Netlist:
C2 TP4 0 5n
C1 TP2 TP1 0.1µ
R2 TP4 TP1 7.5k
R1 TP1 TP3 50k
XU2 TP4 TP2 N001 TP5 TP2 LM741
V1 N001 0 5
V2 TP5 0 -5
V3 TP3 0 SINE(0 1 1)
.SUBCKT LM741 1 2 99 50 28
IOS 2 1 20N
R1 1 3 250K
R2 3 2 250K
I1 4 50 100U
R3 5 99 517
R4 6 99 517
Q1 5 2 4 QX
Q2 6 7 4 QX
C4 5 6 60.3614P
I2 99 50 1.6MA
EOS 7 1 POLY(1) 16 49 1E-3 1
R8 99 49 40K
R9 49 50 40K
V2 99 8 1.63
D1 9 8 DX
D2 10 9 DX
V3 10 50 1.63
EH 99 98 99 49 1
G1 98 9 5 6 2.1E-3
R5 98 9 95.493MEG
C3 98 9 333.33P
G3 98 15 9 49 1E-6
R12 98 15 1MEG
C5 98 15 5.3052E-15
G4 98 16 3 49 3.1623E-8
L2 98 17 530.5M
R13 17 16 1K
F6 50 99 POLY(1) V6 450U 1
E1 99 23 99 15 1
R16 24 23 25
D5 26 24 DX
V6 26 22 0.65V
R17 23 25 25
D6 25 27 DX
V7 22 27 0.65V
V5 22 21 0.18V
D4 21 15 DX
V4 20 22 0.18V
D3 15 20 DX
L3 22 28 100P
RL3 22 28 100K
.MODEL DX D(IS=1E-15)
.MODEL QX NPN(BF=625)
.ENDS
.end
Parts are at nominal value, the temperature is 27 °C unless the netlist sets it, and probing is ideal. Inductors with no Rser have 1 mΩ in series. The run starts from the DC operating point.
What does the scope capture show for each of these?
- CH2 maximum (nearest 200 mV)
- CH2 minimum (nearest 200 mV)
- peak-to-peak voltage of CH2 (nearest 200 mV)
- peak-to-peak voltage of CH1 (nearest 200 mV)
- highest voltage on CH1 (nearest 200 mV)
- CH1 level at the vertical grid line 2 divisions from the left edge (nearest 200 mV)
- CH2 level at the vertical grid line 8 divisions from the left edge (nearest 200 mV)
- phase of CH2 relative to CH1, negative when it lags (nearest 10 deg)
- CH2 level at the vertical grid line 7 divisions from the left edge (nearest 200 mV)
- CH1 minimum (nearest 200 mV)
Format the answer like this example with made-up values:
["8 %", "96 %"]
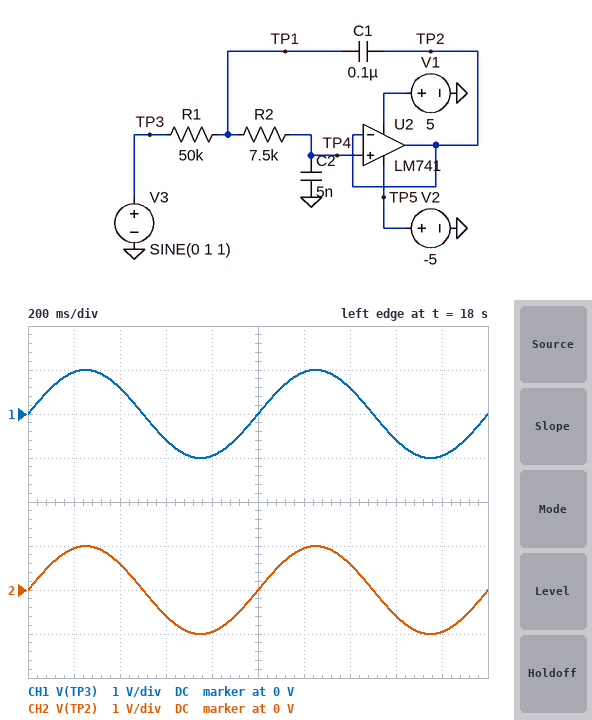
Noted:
["1.0 V", "-1.0 V", "2.0 V", "2.0 V", "1.0 V", "600 mV", "-600 mV", "0 deg", "600 mV", "-1.0 V"]
